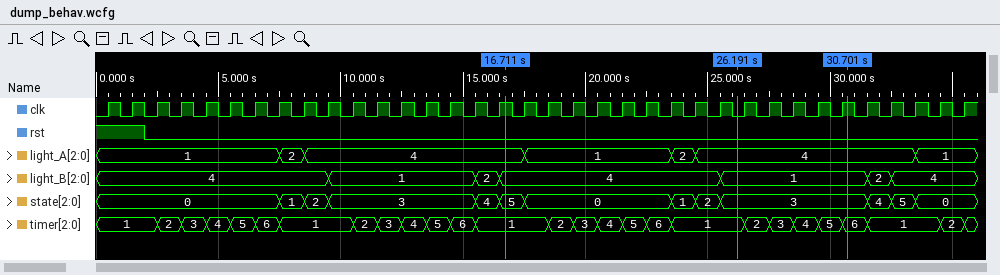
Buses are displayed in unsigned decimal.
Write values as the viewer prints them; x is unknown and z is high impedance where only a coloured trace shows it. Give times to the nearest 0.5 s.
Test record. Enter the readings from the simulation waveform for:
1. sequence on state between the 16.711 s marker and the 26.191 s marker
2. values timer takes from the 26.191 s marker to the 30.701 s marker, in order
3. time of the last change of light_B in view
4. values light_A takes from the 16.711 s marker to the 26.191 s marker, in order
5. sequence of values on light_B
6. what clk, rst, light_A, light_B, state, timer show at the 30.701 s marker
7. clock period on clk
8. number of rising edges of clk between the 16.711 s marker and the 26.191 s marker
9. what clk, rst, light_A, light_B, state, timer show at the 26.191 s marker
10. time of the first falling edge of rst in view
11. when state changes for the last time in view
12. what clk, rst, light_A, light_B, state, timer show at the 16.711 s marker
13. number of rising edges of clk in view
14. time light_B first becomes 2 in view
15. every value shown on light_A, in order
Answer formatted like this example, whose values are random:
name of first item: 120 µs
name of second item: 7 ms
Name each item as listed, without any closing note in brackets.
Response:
sequence on state between the 16.711 s marker and the 26.191 s marker: 5, 0, 1, 2, 3
values timer takes from the 26.191 s marker to the 30.701 s marker, in order: 1, 2, 3, 4, 5, 6
time of the last change of light_B in view: 32.5 s
values light_A takes from the 16.711 s marker to the 26.191 s marker, in order: 4, 1, 2, 4
sequence of values on light_B: 4, 1, 2, 4, 1, 2, 4
what clk, rst, light_A, light_B, state, timer show at the 30.701 s marker: clk=1, rst=0, light_A=4, light_B=1, state=3, timer=6
clock period on clk: 1 s
number of rising edges of clk between the 16.711 s marker and the 26.191 s marker: 9
what clk, rst, light_A, light_B, state, timer show at the 26.191 s marker: clk=0, rst=0, light_A=4, light_B=1, state=3, timer=1
time of the first falling edge of rst in view: 2 s
when state changes for the last time in view: 33.5 s
what clk, rst, light_A, light_B, state, timer show at the 16.711 s marker: clk=1, rst=0, light_A=4, light_B=4, state=5, timer=1
number of rising edges of clk in view: 36
time light_B first becomes 2 in view: 15.5 s
every value shown on light_A, in order: 1, 2, 4, 1, 2, 4, 1
